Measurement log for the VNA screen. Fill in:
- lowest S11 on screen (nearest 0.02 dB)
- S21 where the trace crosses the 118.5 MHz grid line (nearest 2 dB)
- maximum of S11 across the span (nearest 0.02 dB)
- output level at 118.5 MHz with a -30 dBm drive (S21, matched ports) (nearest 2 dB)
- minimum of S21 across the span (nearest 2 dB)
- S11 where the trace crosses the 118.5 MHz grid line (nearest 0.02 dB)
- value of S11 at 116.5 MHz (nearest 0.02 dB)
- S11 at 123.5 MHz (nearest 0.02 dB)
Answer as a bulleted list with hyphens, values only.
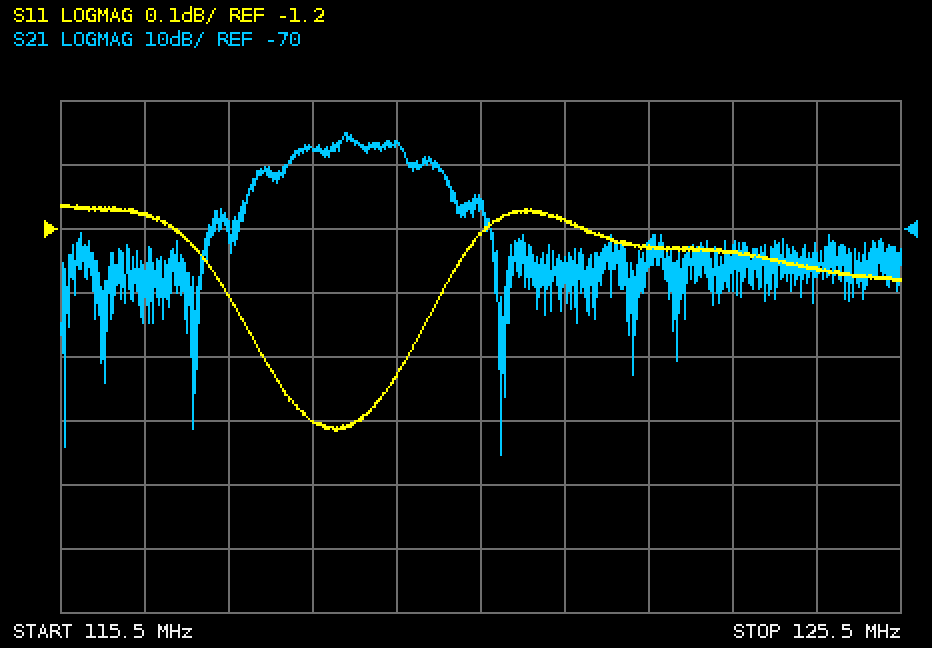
- -1.52 dB
- -58 dB
- -1.16 dB
- -88 dBm
- -106 dB
- -1.50 dB
- -1.18 dB
- -1.24 dB
